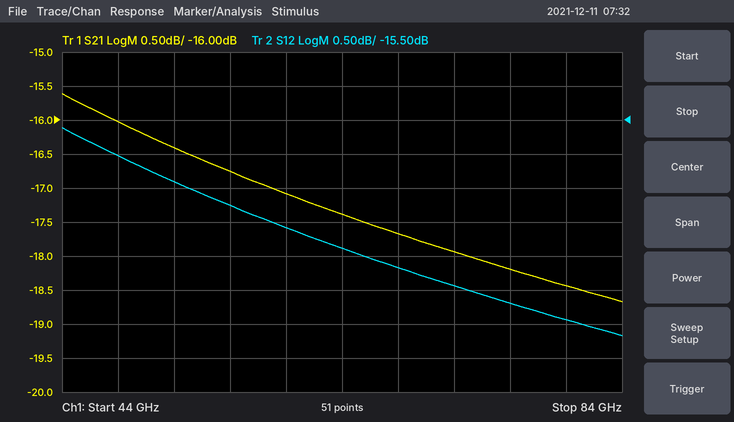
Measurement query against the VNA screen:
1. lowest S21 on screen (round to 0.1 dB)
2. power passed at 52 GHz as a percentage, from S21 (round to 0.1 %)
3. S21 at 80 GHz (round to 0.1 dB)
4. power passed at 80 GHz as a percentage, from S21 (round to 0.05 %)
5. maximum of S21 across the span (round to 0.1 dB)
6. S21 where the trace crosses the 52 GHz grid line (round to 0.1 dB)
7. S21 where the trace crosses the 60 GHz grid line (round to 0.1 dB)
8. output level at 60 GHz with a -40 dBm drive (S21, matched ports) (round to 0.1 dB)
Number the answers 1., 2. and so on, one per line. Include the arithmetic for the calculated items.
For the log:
1. -18.7 dB
2. 10^(-16.4/10) ≈ 2.3 %
3. -18.4 dB
4. 10^(-18.4/10) ≈ 1.45 %
5. -15.6 dB
6. -16.4 dB
7. -17.1 dB
8. -40 dBm + (-17.1 dB) = -57.1 dBm
